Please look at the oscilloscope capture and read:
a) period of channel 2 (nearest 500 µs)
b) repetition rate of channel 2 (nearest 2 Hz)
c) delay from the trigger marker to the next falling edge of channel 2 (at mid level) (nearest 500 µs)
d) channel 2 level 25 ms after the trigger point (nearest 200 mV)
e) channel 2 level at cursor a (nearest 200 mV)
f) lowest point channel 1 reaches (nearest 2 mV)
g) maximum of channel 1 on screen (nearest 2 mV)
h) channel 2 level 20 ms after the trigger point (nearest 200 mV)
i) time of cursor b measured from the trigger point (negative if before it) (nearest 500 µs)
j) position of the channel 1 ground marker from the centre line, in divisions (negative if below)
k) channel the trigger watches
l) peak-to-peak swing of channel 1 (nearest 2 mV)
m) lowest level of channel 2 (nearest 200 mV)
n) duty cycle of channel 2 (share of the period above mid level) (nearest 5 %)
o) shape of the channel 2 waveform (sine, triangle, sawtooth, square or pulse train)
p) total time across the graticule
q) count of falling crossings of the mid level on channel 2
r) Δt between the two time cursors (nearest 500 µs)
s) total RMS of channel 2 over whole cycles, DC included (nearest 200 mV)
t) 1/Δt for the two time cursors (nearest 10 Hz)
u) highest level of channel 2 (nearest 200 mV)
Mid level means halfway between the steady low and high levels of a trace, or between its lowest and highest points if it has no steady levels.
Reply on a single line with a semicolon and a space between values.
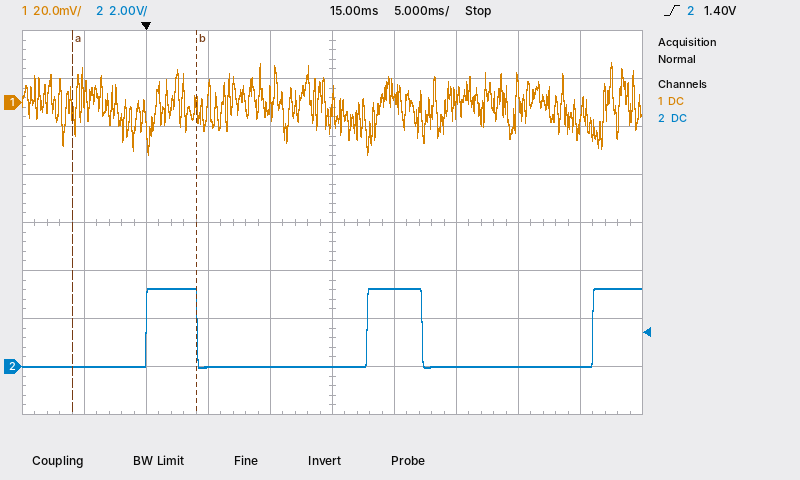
18.0 ms; 56 Hz; 4.0 ms; 0.0 V; 0.0 V; -22 mV; 16 mV; 3.2 V; +4.0 ms; +2.5 div; channel 2; 38 mV; 0.0 V; 25 %; pulse train; 50 ms; 2; 10.0 ms; 1.6 V; 100 Hz; 3.2 V
